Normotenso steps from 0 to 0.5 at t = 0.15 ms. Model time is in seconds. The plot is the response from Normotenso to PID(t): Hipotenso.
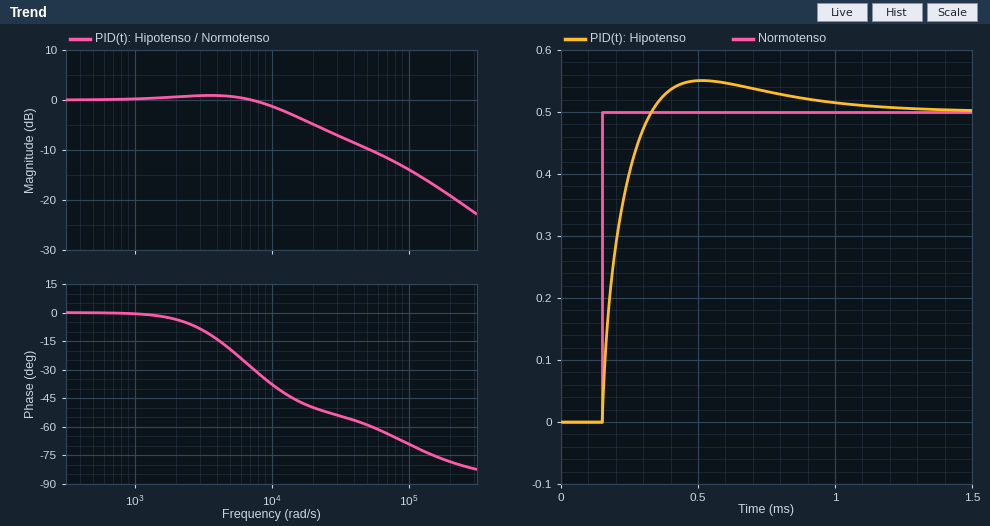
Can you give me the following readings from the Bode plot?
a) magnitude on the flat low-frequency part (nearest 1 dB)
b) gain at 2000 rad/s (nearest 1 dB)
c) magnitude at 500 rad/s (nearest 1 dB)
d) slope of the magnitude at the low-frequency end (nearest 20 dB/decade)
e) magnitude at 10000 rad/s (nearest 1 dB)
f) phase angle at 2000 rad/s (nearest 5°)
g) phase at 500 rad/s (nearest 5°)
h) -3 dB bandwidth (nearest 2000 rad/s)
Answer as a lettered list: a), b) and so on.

a) 0 dB
b) 1 dB
c) 0 dB
d) 0 dB/decade
e) -1 dB
f) -5°
g) 0°
h) 14000 rad/s
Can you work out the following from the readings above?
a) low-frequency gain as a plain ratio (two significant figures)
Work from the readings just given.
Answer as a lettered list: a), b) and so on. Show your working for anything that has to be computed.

a) 10^(0 / 20) = 1.0
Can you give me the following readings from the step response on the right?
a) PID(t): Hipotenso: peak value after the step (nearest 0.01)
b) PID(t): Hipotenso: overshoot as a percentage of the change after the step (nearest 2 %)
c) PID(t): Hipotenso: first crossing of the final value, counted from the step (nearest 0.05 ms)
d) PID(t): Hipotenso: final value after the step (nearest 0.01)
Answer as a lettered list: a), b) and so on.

a) 0.55
b) 10 %
c) 0.20 ms
d) 0.50
